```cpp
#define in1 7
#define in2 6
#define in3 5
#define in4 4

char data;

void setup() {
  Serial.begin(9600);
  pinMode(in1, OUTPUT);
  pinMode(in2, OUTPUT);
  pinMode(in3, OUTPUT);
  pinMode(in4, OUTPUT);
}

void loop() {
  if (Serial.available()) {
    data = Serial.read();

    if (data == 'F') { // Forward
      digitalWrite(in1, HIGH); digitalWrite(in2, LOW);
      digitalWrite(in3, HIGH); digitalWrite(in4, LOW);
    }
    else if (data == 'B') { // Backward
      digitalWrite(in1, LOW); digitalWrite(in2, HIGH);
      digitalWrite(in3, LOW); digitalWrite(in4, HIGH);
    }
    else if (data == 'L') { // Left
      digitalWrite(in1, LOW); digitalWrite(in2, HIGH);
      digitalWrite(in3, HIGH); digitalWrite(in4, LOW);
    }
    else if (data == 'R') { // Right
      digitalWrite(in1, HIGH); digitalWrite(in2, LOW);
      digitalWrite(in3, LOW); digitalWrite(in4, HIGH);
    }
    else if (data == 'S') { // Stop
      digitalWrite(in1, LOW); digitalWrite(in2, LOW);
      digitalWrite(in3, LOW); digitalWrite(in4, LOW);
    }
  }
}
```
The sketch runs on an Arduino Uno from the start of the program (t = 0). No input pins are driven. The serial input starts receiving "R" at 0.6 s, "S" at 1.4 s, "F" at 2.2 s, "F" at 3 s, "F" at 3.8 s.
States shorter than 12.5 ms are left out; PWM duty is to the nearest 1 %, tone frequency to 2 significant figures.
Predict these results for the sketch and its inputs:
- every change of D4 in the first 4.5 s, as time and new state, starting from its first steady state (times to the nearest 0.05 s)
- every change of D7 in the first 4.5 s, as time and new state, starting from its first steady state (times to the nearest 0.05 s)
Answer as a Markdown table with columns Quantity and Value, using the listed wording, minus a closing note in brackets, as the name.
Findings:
| Quantity | Value |
|---|---|
| every change of D4 in the first 4.5 s, as time and new state, starting from its first steady state | 0 s low; 0.6 s high; 1.4 s low |
| every change of D7 in the first 4.5 s, as time and new state, starting from its first steady state | 0 s low; 0.6 s high; 1.4 s low; 2.2 s high |
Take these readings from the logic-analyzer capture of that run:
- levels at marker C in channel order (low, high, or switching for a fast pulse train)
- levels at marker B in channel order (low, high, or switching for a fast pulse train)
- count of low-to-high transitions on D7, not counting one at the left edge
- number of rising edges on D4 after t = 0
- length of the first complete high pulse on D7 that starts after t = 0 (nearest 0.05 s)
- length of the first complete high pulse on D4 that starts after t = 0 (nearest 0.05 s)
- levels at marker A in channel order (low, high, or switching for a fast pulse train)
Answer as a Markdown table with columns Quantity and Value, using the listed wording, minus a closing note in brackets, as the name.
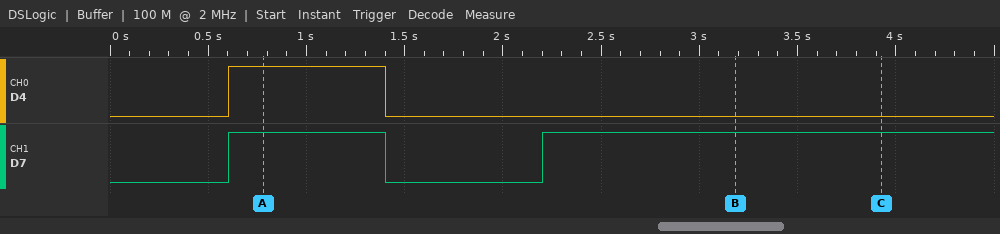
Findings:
| Quantity | Value |
|---|---|
| levels at marker C in channel order | D4 low, D7 high |
| levels at marker B in channel order | D4 low, D7 high |
| count of low-to-high transitions on D7, not counting one at the left edge | 2 |
| number of rising edges on D4 after t = 0 | 1 |
| length of the first complete high pulse on D7 that starts after t = 0 | 0.80 s |
| length of the first complete high pulse on D4 that starts after t = 0 | 0.80 s |
| levels at marker A in channel order | D4 high, D7 high |
